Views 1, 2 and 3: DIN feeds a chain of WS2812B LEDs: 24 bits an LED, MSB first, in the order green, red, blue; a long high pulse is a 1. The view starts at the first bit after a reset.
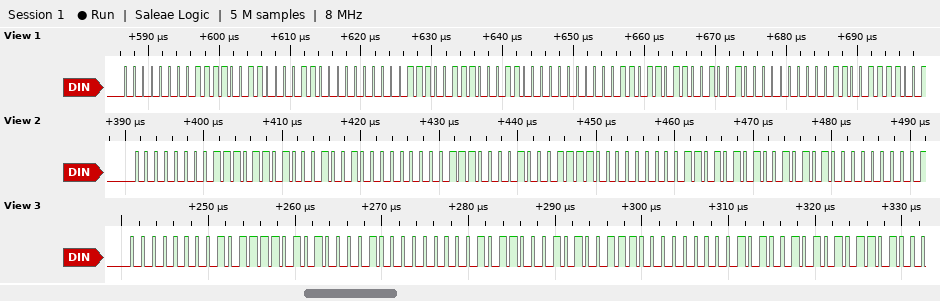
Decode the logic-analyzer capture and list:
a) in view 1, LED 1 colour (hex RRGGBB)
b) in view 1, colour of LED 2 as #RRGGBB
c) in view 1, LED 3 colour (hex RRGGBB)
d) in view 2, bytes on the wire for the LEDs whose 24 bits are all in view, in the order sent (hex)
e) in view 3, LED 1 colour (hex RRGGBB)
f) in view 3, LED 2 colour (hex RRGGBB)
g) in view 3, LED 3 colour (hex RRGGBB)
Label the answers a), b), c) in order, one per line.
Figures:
a) #F3000C
b) #E70018
c) #DB0024
d) 00 ED 12 00 E1 1E 00 D5 2A
e) #BD0042
f) #B1004E
g) #A5005A
